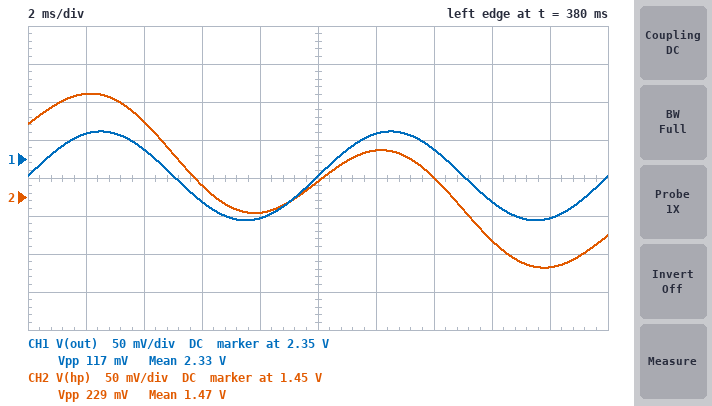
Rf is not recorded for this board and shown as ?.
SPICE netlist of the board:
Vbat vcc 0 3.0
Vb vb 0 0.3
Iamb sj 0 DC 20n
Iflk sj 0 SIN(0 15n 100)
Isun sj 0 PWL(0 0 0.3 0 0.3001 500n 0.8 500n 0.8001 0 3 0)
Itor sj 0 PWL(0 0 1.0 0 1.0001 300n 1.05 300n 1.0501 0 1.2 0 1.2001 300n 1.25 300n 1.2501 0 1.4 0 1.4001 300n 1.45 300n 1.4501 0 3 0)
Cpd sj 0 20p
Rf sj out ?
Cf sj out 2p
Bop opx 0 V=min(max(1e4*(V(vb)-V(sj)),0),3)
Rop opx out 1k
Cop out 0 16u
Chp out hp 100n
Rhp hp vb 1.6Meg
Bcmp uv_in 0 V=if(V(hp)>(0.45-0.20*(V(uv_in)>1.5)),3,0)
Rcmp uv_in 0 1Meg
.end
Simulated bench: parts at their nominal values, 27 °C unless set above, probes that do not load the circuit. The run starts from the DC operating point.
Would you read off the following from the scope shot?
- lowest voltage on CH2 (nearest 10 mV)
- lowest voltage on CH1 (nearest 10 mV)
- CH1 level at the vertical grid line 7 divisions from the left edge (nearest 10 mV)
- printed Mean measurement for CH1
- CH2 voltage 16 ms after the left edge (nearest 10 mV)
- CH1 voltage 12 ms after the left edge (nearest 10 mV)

1.36 V
2.27 V
2.36 V
2.33 V
1.39 V
2.38 V
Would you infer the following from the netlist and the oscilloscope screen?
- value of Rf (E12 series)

3.9 MΩ
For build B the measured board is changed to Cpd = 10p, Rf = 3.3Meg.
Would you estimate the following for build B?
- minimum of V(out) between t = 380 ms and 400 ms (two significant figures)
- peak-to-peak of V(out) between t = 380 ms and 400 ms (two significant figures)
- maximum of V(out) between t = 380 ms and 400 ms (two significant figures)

2.0 V
99 mV
2.1 V
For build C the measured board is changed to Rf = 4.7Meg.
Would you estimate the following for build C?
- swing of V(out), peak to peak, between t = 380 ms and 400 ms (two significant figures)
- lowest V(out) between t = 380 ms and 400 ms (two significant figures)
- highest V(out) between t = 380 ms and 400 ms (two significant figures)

110 mV
2.7 V
2.8 V
